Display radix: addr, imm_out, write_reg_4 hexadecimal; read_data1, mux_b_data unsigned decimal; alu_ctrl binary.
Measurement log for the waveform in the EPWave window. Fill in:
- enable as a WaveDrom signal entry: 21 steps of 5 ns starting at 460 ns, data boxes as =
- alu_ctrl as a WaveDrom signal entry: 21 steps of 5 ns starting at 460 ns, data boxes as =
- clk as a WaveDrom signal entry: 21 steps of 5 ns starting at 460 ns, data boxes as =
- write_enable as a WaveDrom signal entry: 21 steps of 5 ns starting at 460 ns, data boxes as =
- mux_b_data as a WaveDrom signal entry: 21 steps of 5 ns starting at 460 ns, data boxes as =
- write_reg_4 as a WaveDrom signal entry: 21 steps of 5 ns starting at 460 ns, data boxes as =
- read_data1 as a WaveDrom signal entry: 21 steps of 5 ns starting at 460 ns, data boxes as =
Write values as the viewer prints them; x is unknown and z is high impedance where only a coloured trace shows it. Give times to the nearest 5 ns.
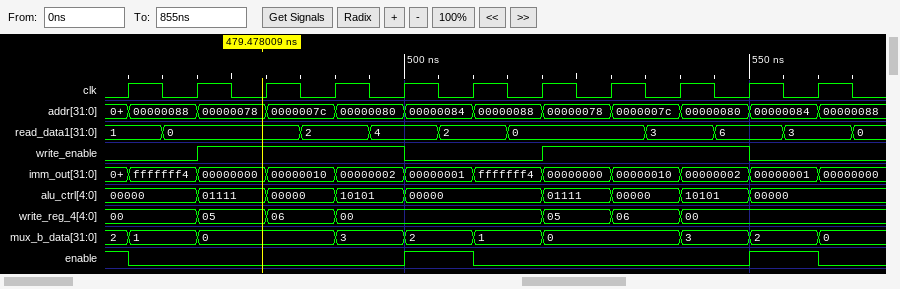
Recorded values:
{name: 'enable', wave: '0.......1.0.......1.0'}
{name: 'alu_ctrl', wave: '=.=.=.=.=...=.=.=.=..', data: '00000 01111 00000 10101 00000 01111 00000 10101 00000'}
{name: 'clk', wave: '101010101010101010101'}
{name: 'write_enable', wave: '0.1.....0...1.....0..'}
{name: 'mux_b_data', wave: '=.=...=.=.=.=...=.=.=', data: '1 0 3 2 1 0 3 2 0'}
{name: 'write_reg_4', wave: '=.=.=.=.....=.=.=....', data: '00 05 06 00 05 06 00'}
{name: 'read_data1', wave: '==...=.=.=.=...=.=.=.', data: '1 0 2 4 2 0 3 6 3'}
